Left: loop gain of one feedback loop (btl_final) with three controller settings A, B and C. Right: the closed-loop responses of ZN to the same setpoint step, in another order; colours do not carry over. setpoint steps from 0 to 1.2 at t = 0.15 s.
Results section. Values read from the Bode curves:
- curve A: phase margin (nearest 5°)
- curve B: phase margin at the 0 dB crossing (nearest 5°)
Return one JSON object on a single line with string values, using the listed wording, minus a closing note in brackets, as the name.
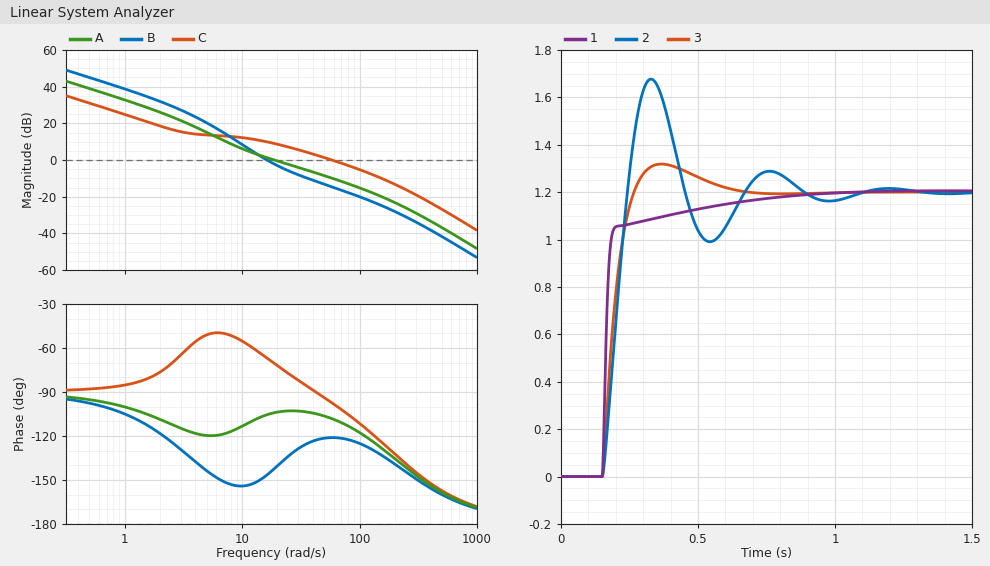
{"curve A: phase margin": "75°", "curve B: phase margin at the 0 dB crossing": "35°"}
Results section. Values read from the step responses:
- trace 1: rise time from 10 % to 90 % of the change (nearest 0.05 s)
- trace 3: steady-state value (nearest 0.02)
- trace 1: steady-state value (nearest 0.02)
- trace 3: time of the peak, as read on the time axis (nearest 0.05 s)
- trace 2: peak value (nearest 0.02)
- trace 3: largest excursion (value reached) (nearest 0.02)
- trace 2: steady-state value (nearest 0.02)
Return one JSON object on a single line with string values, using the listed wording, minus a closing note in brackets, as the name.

{"trace 1: rise time from 10 % to 90 % of the change": "0.15 s", "trace 3: steady-state value": "1.20", "trace 1: steady-state value": "1.20", "trace 3: time of the peak, as read on the time axis": "0.35 s", "trace 2: peak value": "1.68", "trace 3: largest excursion (value reached)": "1.32", "trace 2: steady-state value": "1.20"}
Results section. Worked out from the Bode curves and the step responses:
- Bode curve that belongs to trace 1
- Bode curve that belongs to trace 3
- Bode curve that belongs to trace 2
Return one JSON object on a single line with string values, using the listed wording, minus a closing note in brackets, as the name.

{"Bode curve that belongs to trace 1": "C", "Bode curve that belongs to trace 3": "A", "Bode curve that belongs to trace 2": "B"}
